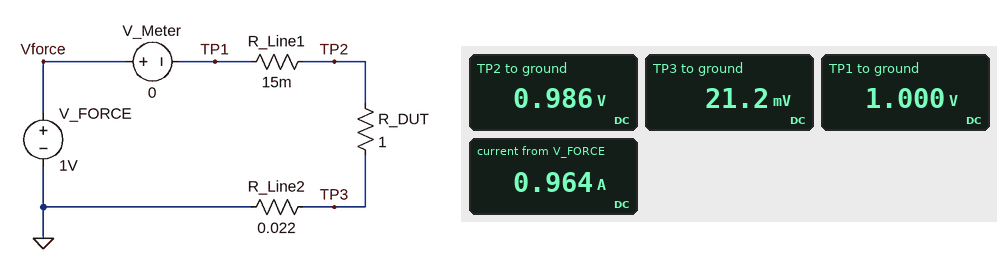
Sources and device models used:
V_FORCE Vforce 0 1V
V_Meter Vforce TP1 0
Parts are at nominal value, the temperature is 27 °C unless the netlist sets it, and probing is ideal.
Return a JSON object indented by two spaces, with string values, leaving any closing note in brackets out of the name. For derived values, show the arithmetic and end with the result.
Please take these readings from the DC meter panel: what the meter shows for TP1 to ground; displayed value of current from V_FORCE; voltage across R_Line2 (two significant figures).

{
  "what the meter shows for TP1 to ground": "1.000 V",
  "displayed value of current from V_FORCE": "0.964 A",
  "voltage across R_Line2": "21.2 mV = 21 mV"
}
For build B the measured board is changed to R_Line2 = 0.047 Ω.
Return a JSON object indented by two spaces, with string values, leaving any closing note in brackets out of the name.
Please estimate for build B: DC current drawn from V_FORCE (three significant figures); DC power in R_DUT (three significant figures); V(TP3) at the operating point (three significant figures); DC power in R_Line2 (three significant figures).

{
  "DC current drawn from V_FORCE": "942 mA",
  "DC power in R_DUT": "887 mW",
  "V(TP3) at the operating point": "44.3 mV",
  "DC power in R_Line2": "41.7 mW"
}
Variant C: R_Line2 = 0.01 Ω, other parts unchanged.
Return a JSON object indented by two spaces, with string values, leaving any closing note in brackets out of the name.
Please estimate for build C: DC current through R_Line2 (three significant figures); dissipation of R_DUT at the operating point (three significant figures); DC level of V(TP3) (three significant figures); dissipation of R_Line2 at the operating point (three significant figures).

{
  "DC current through R_Line2": "976 mA",
  "dissipation of R_DUT at the operating point": "952 mW",
  "DC level of V(TP3)": "9.76 mV",
  "dissipation of R_Line2 at the operating point": "9.52 mW"
}
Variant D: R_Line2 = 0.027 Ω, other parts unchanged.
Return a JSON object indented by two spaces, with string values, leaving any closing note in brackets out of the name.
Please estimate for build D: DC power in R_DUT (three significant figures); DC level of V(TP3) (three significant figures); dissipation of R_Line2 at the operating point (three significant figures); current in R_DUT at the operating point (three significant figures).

{
  "DC power in R_DUT": "921 mW",
  "DC level of V(TP3)": "25.9 mV",
  "dissipation of R_Line2 at the operating point": "24.9 mW",
  "current in R_DUT at the operating point": "960 mA"
}
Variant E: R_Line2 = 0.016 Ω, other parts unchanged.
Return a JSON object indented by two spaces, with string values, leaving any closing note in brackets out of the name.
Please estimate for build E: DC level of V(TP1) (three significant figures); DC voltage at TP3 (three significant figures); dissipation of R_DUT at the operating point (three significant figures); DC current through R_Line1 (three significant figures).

{
  "DC level of V(TP1)": "1.00 V",
  "DC voltage at TP3": "15.5 mV",
  "dissipation of R_DUT at the operating point": "941 mW",
  "DC current through R_Line1": "970 mA"
}
